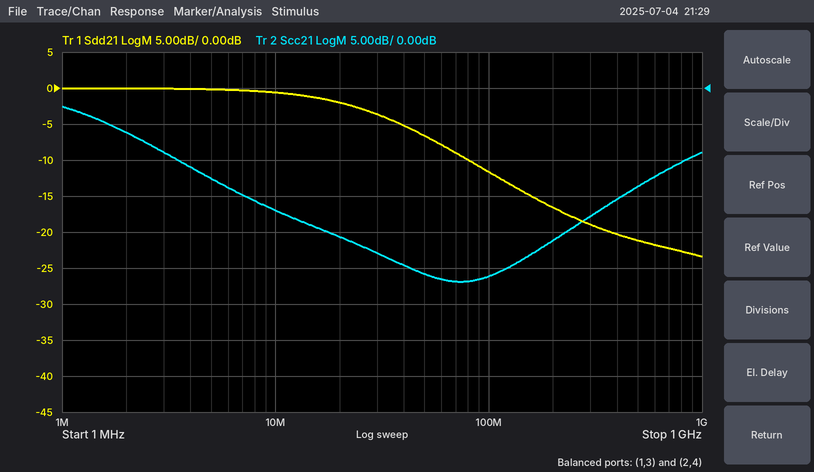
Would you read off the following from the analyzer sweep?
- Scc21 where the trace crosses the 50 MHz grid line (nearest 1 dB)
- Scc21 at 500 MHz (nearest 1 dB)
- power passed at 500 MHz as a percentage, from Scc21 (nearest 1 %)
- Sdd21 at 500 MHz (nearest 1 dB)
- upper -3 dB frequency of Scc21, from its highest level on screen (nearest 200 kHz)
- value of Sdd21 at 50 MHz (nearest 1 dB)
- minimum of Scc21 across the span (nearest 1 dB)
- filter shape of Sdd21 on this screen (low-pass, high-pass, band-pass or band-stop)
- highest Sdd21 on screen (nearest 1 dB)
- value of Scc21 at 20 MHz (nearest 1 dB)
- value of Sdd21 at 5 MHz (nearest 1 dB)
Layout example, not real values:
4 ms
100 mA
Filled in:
-26 dB
-14 dB
4 %
-21 dB
1.8 MHz
-7 dB
-27 dB
low-pass
0 dB
-21 dB
0 dB
